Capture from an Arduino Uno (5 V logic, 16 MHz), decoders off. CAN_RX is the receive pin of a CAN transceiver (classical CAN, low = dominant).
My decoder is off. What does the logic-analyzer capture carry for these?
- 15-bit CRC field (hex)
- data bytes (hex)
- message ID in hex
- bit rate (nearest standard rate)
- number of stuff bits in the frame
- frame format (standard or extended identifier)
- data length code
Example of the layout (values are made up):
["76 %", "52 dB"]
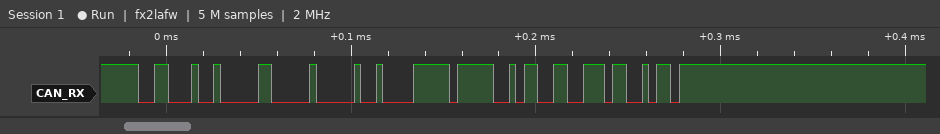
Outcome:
["0x6765", "00 21 FF AC", "0x312", "250 kbit/s", "5", "standard", "4"]
